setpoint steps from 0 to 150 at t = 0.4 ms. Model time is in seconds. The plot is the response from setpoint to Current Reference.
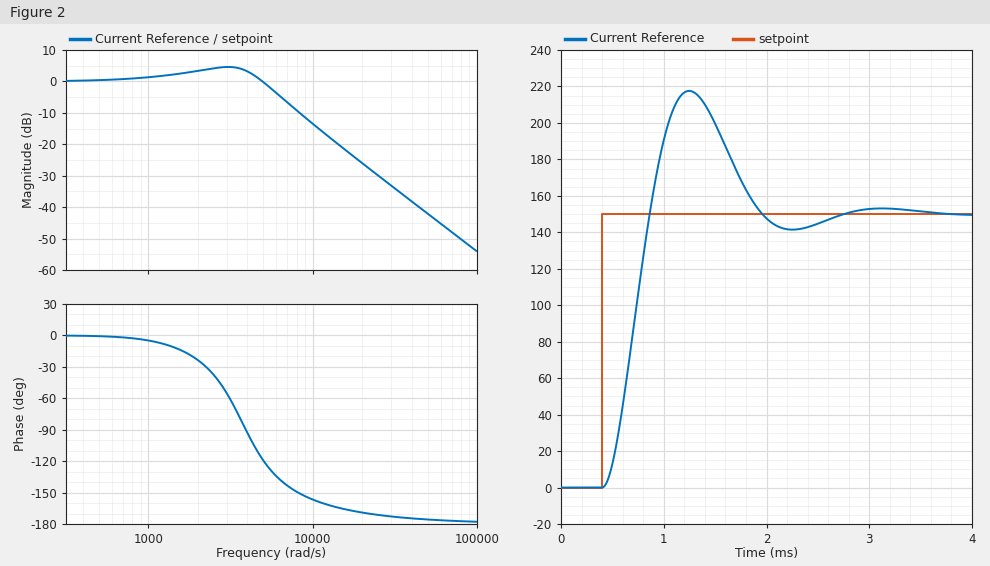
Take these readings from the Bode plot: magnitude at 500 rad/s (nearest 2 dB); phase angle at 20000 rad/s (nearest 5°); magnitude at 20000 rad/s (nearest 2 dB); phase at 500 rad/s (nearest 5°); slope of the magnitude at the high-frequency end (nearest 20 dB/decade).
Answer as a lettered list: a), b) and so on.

a) 0 dB
b) -170°
c) -26 dB
d) 0°
e) -40 dB/decade
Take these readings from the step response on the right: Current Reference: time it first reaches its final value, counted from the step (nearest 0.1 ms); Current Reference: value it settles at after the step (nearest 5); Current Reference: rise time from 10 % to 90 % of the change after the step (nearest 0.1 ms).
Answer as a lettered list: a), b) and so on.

a) 0.5 ms
b) 150
c) 0.3 ms
